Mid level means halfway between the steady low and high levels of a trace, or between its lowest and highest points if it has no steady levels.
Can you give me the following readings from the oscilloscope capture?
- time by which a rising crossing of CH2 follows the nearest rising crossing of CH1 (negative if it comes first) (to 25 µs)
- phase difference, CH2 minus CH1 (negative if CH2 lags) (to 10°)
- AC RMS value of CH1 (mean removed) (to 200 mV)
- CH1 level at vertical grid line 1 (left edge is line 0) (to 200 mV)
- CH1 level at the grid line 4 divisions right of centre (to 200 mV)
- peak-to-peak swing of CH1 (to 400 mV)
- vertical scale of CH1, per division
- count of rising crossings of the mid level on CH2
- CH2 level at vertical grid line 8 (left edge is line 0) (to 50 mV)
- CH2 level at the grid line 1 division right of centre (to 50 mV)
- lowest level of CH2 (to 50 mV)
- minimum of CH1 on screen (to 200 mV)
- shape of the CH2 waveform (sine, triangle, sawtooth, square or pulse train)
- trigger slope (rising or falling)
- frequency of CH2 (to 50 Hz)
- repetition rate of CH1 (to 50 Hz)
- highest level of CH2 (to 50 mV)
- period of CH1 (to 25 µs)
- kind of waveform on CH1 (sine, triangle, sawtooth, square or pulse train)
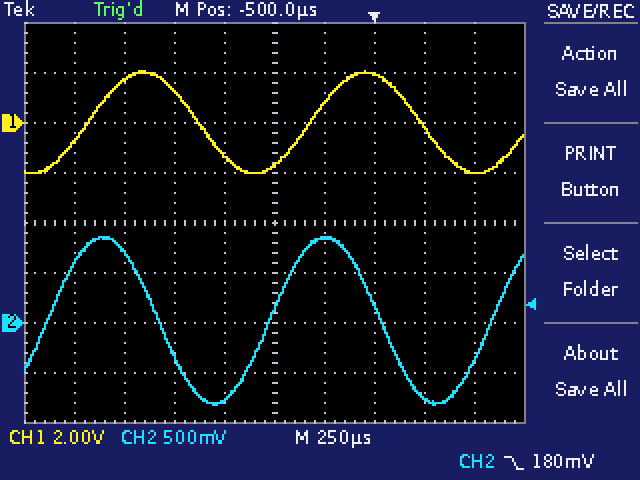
-200 µs
+70°
1.4 V
-800 mV
-2.0 V
4.0 V
2 V
3
-750 mV
850 mV
-800 mV
-2.0 V
sine
falling
900 Hz
900 Hz
850 mV
1.100 ms
sine
